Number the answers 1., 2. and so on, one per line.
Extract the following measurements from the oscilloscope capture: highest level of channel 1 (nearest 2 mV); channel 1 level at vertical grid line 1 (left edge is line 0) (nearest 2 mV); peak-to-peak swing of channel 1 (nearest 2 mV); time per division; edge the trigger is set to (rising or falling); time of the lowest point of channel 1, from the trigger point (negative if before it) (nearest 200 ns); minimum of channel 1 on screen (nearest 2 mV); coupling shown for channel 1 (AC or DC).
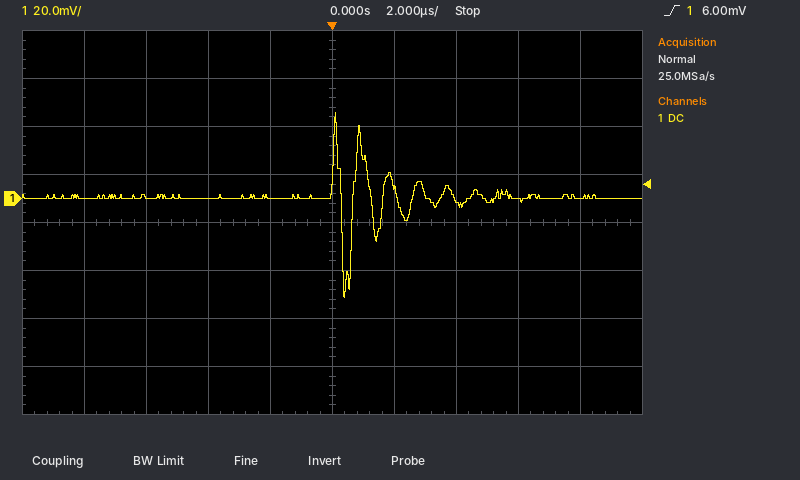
1. 36 mV
2. 0 mV
3. 78 mV
4. 2 µs
5. rising
6. +400 ns
7. -42 mV
8. DC
